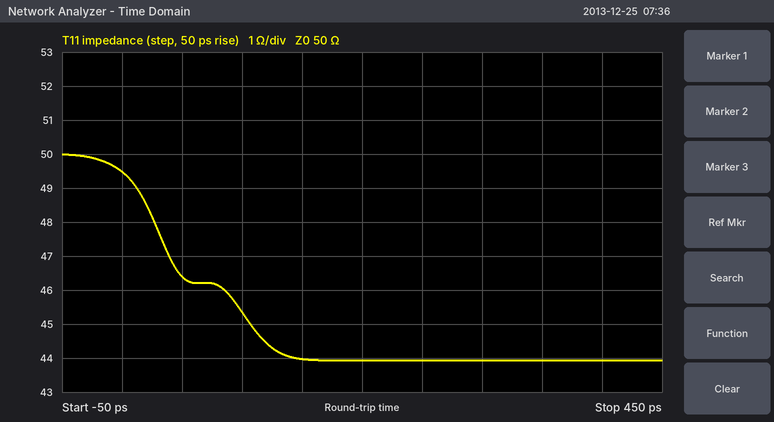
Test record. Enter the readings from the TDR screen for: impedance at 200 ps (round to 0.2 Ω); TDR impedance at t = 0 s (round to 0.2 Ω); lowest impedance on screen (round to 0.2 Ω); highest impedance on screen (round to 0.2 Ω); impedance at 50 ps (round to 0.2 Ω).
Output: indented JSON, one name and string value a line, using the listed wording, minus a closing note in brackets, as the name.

{
  "impedance at 200 ps": "44.0 Ω",
  "TDR impedance at t = 0 s": "49.4 Ω",
  "lowest impedance on screen": "44.0 Ω",
  "highest impedance on screen": "50.0 Ω",
  "impedance at 50 ps": "46.4 Ω"
}
